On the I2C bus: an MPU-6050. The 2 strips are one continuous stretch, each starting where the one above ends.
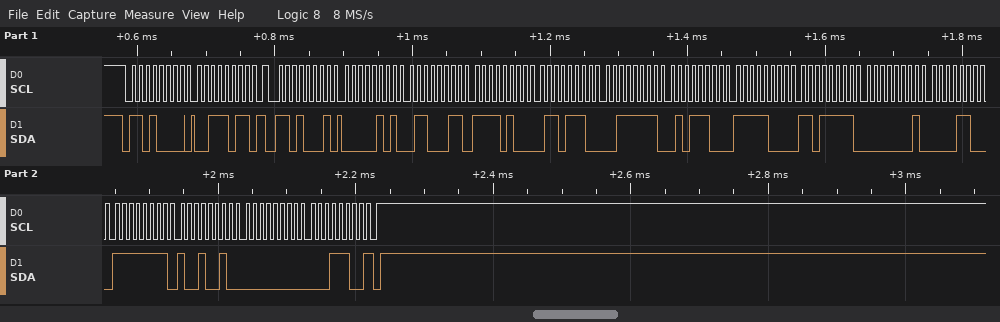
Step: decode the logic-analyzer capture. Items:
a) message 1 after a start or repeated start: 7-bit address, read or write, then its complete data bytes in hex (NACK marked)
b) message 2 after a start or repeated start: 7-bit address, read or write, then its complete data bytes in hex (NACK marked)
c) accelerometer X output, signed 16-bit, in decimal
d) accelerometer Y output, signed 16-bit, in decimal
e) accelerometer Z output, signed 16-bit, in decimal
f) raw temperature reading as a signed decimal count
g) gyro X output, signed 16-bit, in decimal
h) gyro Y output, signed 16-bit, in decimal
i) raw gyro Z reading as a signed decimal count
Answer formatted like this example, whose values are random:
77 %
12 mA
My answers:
0x68 write: 3B
0x68 read: 05 63 F4 6E 3F 5C F8 DF 01 0C FF 92 00 1C NACK
1379
-2962
16220
-1825
268
-110
28
